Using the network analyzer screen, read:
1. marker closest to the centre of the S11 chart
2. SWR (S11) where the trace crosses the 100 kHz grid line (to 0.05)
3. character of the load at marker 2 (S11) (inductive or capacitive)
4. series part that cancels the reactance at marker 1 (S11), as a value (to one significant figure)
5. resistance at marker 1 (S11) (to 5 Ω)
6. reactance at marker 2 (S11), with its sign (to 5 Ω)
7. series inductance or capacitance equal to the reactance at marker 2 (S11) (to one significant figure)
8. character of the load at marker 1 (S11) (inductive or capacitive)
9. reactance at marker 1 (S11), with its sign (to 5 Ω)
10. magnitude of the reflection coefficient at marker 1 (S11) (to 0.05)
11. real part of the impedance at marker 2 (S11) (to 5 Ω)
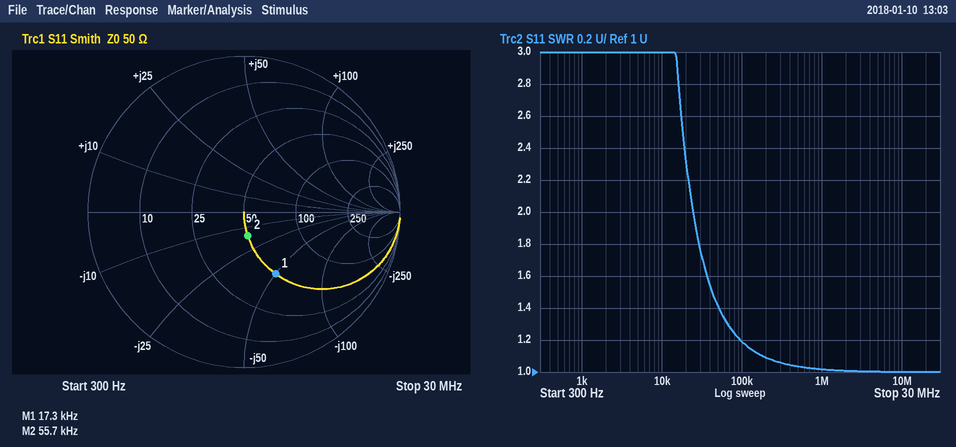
marker 2
1.20
capacitive
500 µH
50 Ω
-15 Ω
200 nF
capacitive
-50 Ω
0.45
50 Ω
